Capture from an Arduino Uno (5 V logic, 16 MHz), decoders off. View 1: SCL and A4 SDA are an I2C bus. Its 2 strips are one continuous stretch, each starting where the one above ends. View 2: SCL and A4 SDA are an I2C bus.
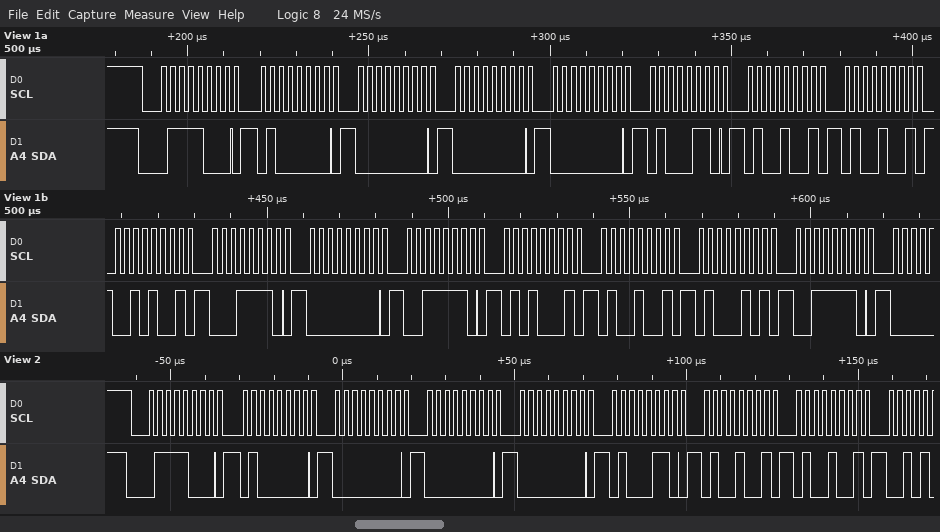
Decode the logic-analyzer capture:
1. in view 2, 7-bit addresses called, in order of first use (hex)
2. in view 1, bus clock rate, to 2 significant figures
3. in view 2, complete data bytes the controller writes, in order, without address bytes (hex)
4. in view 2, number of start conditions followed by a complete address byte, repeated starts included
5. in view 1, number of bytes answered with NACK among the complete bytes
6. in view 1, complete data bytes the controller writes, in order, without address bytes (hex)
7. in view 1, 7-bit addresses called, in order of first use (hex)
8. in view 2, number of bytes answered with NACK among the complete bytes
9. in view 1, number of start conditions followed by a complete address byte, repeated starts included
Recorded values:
0x3C
400 kHz
40 00 00 00 46 49 49
1
0
40 00 00 00 46 49 49 29 1E 00 3E 51 49 45 3E
0x3C
0
1
